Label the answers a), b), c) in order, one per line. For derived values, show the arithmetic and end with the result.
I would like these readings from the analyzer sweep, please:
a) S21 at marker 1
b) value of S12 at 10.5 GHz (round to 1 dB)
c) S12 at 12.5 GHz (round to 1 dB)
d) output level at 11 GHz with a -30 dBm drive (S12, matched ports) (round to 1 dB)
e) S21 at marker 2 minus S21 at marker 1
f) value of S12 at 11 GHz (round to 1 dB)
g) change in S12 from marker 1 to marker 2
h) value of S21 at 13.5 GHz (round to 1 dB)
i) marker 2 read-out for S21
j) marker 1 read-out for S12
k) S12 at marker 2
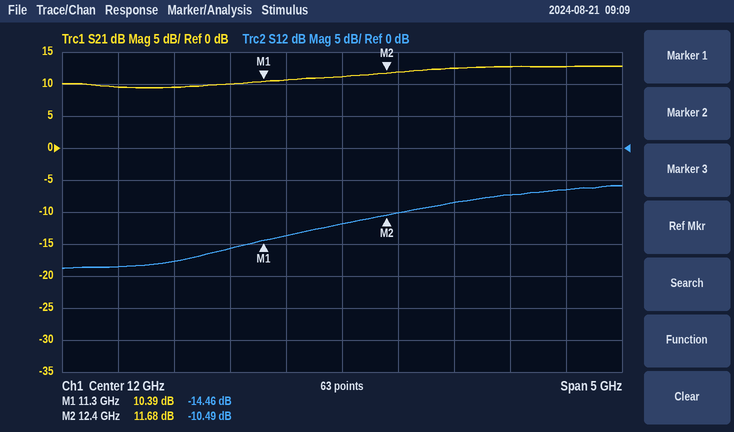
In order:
a) 10.39 dB
b) -18 dB
c) -10 dB
d) -30 dBm + (-16 dB) = -46 dBm
e) 11.68 − (10.39) = 1.29 dB
f) -16 dB
g) -10.49 − (-14.46) = 3.97 dB
h) 13 dB
i) 11.68 dB
j) -14.46 dB
k) -10.49 dB
